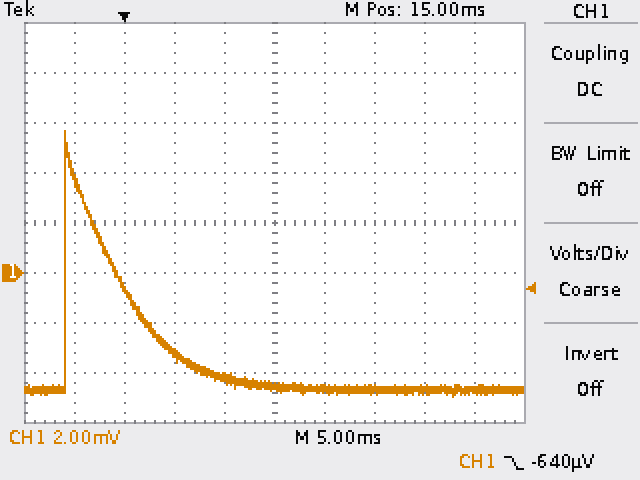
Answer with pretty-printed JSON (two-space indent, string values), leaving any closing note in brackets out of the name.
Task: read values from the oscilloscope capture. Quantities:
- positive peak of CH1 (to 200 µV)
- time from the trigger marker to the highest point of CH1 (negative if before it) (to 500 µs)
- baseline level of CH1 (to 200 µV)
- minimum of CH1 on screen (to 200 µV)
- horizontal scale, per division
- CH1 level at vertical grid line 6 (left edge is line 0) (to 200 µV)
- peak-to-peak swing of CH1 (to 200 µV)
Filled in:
{
  "positive peak of CH1": "5.6 mV",
  "time from the trigger marker to the highest point of CH1 (negative if before it)": "-6.0 ms",
  "baseline level of CH1": "-4.6 mV",
  "minimum of CH1 on screen": "-5.0 mV",
  "horizontal scale, per division": "5 ms",
  "CH1 level at vertical grid line 6 (left edge is line 0)": "-4.6 mV",
  "peak-to-peak swing of CH1": "10.6 mV"
}
